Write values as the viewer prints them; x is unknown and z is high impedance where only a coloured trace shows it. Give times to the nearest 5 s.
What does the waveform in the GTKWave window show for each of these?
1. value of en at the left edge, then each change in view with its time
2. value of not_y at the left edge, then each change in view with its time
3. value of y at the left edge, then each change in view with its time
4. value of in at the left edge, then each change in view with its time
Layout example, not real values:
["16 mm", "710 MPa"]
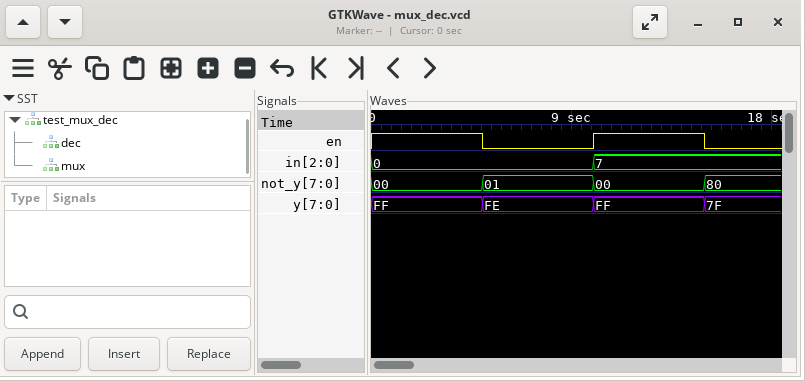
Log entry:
["1, 0 at 5 s, 1 at 10 s, 0 at 15 s", "00, 01 at 5 s, 00 at 10 s, 80 at 15 s", "FF, FE at 5 s, FF at 10 s, 7F at 15 s", "0, 7 at 10 s"]
